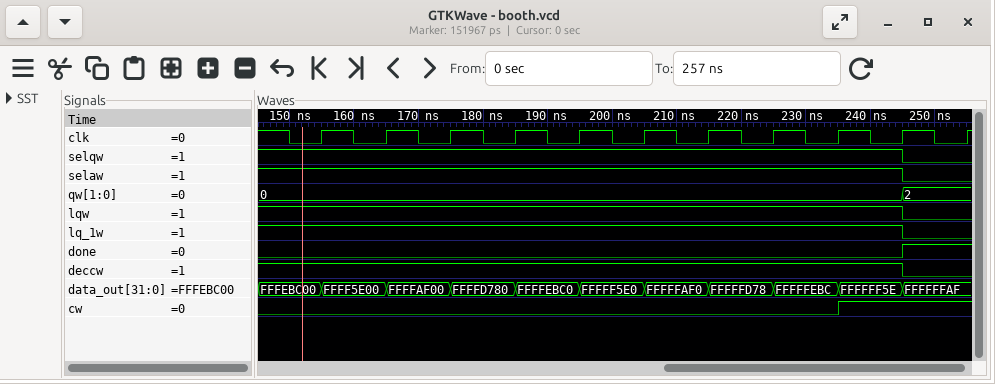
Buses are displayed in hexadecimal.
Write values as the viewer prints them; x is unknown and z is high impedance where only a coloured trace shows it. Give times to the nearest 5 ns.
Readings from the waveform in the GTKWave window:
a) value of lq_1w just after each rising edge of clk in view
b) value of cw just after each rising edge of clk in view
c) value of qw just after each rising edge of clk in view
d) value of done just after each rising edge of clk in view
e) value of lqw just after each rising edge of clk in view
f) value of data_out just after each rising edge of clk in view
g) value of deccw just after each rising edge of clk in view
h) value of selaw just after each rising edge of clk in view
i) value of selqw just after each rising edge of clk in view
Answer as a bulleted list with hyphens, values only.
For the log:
- 1 1 1 1 1 1 1 1 1 0 0
- 0 0 0 0 0 0 0 0 1 1 1
- 0, 0, 0, 0, 0, 0, 0, 0, 0, 2, 2
- 0 0 0 0 0 0 0 0 0 1 1
- 1 1 1 1 1 1 1 1 1 0 0
- FFFF5E00, FFFFAF00, FFFFD780, FFFFEBC0, FFFFF5E0, FFFFFAF0, FFFFFD78, FFFFFEBC, FFFFFF5E, FFFFFFAF, FFFFFFAF
- 1 1 1 1 1 1 1 1 1 0 0
- 1 1 1 1 1 1 1 1 1 0 0
- 1 1 1 1 1 1 1 1 1 0 0
